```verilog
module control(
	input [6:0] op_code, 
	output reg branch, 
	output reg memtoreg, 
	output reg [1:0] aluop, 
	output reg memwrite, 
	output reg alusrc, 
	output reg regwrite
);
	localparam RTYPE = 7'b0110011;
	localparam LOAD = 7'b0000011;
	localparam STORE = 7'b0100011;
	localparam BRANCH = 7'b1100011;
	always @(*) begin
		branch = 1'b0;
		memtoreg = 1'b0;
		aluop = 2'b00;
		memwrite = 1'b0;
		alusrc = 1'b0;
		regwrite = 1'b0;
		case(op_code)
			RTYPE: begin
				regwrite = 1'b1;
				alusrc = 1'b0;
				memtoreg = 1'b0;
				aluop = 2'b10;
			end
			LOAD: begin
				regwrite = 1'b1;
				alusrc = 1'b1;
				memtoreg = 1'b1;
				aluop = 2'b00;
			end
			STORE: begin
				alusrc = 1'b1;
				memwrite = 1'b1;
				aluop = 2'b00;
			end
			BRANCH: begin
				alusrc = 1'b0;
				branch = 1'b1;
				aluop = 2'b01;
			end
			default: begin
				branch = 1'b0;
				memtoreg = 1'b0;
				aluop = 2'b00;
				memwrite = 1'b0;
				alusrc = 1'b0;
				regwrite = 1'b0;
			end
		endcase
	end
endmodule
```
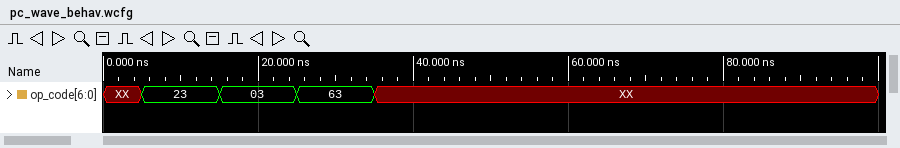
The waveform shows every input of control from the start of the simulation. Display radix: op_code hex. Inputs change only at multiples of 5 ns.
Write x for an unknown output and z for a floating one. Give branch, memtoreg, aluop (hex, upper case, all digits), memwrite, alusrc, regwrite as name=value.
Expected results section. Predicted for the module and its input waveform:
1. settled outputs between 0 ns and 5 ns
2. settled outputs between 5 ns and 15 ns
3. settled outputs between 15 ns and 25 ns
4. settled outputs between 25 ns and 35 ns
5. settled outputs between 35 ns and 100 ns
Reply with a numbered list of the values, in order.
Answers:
1. branch=x, memtoreg=x, aluop=x, memwrite=x, alusrc=x, regwrite=x
2. branch=0, memtoreg=0, aluop=0, memwrite=1, alusrc=1, regwrite=0
3. branch=0, memtoreg=1, aluop=0, memwrite=0, alusrc=1, regwrite=1
4. branch=1, memtoreg=0, aluop=1, memwrite=0, alusrc=0, regwrite=0
5. branch=0, memtoreg=0, aluop=0, memwrite=0, alusrc=0, regwrite=0
